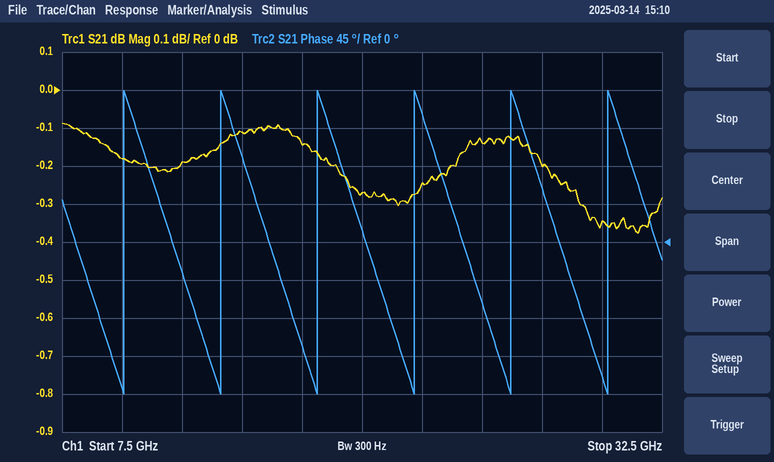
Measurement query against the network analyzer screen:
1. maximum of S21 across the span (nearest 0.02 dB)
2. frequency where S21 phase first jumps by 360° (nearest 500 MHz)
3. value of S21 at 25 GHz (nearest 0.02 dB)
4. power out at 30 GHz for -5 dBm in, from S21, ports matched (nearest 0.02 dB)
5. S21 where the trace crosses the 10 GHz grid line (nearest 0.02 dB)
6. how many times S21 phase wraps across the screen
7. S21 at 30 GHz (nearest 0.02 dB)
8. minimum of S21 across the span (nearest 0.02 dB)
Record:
-0.08 dB
10.0 GHz
-0.14 dB
-5.34 dBm
-0.18 dB
6
-0.34 dB
-0.38 dB
